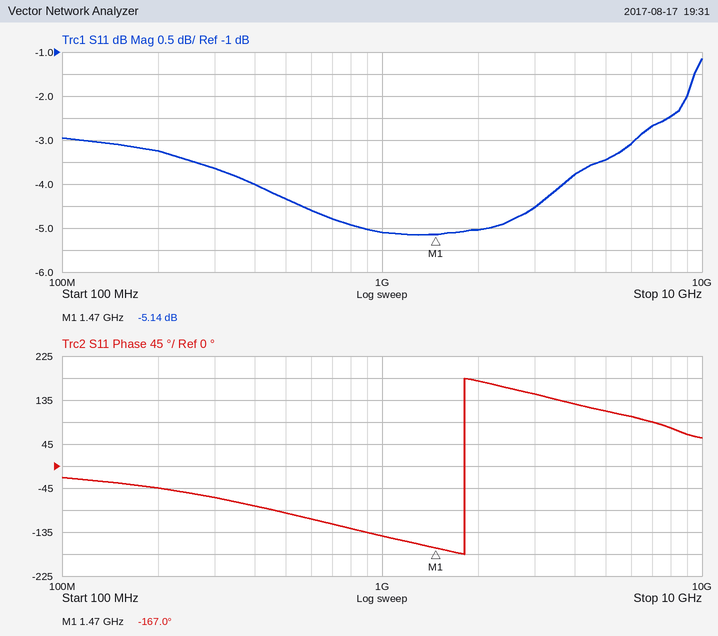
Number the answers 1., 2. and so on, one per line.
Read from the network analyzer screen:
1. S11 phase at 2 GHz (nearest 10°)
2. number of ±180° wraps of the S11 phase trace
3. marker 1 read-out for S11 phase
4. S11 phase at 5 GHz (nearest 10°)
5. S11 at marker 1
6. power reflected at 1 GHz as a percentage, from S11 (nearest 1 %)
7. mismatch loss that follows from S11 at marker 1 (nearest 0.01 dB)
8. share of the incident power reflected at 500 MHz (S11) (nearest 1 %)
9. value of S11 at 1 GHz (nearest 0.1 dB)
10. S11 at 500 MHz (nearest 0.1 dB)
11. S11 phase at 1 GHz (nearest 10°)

1. 170°
2. 1
3. -167.0°
4. 110°
5. -5.14 dB
6. 31 %
7. 1.59 dB
8. 37 %
9. -5.1 dB
10. -4.3 dB
11. -140°
